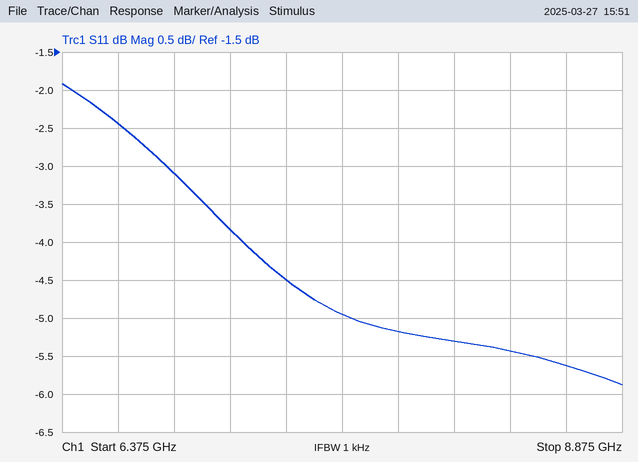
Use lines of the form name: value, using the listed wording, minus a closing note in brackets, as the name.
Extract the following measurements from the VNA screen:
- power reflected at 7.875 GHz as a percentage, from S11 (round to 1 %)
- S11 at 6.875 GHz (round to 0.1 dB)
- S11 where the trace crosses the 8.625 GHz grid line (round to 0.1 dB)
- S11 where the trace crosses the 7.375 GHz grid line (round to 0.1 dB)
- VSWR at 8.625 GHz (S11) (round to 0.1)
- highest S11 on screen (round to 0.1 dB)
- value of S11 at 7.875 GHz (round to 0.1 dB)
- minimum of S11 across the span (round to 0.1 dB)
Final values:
power reflected at 7.875 GHz as a percentage, from S11: 30 %
S11 at 6.875 GHz: -3.1 dB
S11 where the trace crosses the 8.625 GHz grid line: -5.6 dB
S11 where the trace crosses the 7.375 GHz grid line: -4.5 dB
VSWR at 8.625 GHz (S11): 3.2
highest S11 on screen: -1.9 dB
value of S11 at 7.875 GHz: -5.2 dB
minimum of S11 across the span: -5.9 dB
